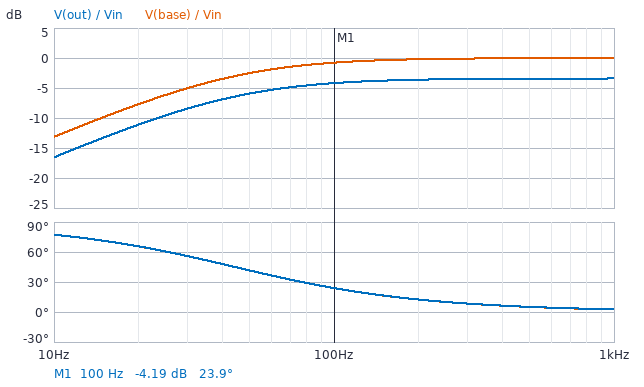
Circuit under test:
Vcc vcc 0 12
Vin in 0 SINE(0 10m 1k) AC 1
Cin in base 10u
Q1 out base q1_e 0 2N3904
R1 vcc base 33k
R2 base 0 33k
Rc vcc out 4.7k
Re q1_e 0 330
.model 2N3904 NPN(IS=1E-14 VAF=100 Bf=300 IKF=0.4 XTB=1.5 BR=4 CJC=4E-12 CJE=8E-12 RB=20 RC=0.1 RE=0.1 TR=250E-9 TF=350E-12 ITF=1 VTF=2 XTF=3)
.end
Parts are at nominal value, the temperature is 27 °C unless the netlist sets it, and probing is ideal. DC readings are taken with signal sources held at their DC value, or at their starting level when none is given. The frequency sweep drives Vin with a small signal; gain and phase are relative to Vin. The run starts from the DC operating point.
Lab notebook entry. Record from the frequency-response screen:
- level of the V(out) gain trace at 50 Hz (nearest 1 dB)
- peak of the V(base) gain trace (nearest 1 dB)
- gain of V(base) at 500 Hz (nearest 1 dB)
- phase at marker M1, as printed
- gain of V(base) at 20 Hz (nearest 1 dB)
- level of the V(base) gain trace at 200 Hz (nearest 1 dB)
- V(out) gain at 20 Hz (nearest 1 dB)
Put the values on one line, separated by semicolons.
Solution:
-6 dB; 0 dB; 0 dB; 23.9 deg; -8 dB; 0 dB; -11 dB
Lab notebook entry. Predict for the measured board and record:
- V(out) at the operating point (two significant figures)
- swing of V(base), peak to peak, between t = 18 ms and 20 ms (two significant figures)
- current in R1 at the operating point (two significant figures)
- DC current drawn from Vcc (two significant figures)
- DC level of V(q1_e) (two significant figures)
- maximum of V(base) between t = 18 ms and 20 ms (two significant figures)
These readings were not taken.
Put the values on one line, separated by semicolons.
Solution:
900 mV; 20 mV; 320 µA; 2.7 mA; 870 mV; 1.6 V
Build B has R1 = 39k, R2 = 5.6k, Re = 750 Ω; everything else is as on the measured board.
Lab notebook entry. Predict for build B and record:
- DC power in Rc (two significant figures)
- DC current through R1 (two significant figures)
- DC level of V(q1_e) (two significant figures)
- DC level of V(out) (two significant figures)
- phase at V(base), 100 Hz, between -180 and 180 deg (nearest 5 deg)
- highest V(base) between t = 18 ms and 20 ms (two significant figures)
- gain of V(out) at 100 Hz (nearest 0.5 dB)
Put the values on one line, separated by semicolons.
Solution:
5.8 mW; 270 µA; 830 mV; 6.8 V; 0 deg; 1.5 V; 15.5 dB
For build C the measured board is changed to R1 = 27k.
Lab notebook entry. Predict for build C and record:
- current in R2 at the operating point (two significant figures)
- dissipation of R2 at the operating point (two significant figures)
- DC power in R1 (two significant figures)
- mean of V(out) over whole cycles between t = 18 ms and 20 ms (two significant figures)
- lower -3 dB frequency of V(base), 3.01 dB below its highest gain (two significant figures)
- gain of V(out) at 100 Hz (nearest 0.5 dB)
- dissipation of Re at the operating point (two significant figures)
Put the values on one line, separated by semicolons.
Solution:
48 µA; 76 µW; 4.0 mW; 920 mV; 45 Hz; -3.5 dB; 2.4 mW
